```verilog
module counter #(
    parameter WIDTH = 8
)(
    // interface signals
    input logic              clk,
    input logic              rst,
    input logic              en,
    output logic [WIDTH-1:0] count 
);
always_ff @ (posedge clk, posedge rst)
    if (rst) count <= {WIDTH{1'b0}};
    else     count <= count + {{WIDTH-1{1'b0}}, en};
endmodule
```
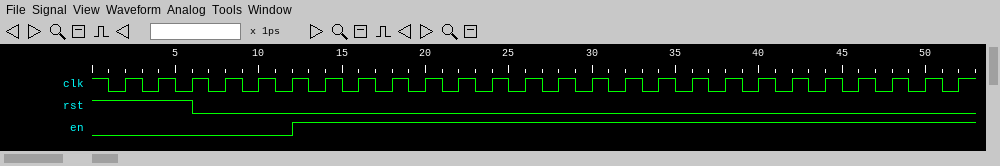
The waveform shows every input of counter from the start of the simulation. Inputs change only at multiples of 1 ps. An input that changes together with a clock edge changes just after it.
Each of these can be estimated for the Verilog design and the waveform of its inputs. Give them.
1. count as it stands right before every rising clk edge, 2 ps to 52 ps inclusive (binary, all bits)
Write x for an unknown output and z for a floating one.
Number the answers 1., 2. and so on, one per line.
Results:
1. 00000000, 00000000, 00000000, 00000000, 00000000, 00000000, 00000000, 00000001, 00000010, 00000011, 00000100, 00000101, 00000110, 00000111, 00001000, 00001001, 00001010, 00001011, 00001100, 00001101, 00001110, 00001111, 00010000, 00010001, 00010010, 00010011
